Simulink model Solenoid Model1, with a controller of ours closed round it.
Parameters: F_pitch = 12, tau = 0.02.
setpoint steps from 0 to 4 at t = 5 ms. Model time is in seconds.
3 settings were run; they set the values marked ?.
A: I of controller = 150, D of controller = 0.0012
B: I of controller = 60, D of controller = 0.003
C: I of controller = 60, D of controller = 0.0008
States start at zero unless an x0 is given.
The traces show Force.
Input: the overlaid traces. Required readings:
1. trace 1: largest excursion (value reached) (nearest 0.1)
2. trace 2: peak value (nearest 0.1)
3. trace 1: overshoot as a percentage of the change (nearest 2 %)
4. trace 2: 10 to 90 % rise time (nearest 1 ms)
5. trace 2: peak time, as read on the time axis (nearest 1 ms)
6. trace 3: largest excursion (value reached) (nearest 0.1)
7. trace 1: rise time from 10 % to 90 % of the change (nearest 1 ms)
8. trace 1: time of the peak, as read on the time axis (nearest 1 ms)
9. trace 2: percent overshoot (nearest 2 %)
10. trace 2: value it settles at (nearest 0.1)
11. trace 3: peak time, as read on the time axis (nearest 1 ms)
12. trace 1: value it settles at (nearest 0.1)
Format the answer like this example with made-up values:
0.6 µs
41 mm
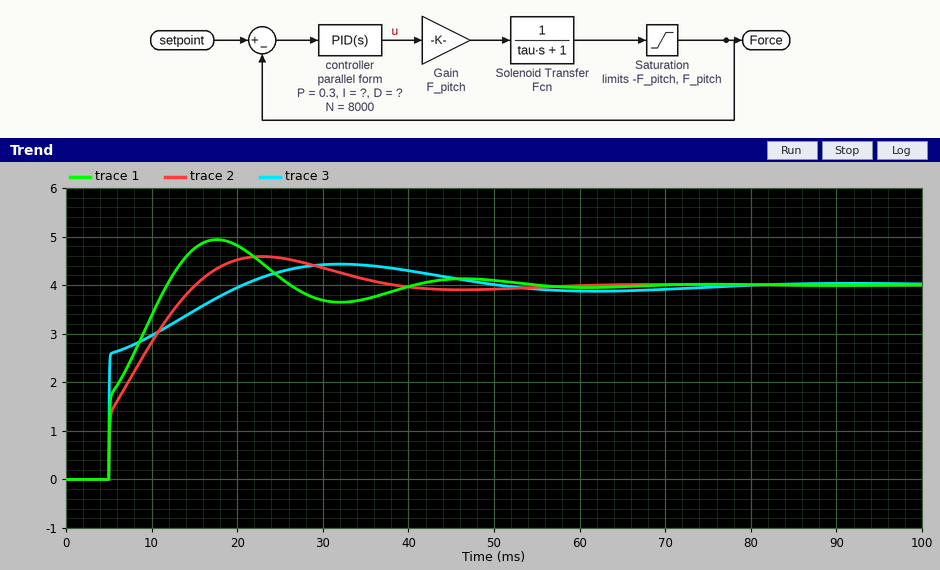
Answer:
4.9
4.6
24 %
8 ms
23 ms
4.4
6 ms
18 ms
14 %
4.0
32 ms
4.0
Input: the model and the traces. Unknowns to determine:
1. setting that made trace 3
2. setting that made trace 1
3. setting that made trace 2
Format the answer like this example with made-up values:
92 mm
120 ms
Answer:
B
A
C
